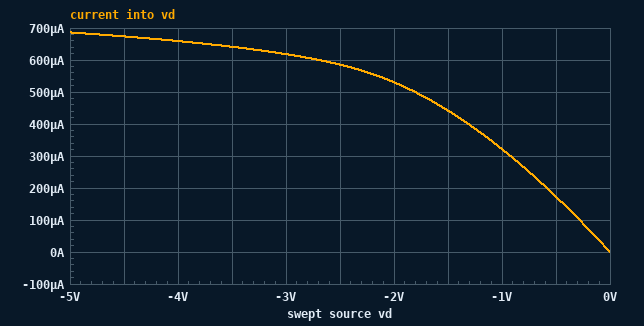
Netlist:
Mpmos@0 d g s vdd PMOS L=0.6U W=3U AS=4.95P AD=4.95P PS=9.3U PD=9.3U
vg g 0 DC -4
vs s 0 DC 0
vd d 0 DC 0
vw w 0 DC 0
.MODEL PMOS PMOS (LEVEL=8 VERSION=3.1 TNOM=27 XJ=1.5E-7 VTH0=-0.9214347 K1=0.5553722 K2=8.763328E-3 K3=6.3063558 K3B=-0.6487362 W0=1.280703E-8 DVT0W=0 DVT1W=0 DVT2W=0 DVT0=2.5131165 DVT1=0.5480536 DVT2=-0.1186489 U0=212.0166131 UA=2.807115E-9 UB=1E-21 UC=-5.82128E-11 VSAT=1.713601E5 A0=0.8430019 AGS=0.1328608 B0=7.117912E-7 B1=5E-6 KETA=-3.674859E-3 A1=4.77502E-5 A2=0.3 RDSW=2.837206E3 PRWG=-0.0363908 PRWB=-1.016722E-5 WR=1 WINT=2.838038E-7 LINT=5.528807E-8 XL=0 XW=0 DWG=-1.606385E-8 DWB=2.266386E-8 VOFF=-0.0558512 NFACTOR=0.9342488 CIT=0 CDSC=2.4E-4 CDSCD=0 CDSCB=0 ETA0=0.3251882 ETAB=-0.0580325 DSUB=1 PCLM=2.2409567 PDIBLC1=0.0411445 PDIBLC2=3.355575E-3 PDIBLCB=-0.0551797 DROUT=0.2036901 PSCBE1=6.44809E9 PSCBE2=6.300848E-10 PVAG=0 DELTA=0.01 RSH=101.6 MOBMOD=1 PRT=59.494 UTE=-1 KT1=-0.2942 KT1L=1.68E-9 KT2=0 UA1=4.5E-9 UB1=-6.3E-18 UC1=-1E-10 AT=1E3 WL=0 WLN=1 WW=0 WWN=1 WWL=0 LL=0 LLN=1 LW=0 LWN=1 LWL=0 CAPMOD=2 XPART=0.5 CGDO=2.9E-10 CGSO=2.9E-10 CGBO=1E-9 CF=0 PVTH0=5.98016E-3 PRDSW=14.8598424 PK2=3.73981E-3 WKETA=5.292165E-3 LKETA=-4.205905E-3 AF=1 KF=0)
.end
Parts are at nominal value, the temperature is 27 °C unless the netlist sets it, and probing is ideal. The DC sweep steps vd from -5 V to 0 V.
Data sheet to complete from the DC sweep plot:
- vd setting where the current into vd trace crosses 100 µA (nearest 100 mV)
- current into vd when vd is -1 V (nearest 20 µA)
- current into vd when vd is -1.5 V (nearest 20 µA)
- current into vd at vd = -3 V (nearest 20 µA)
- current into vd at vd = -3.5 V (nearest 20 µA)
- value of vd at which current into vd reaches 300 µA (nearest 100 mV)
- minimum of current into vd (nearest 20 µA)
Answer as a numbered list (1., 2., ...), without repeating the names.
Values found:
1. -300 mV
2. 320 µA
3. 440 µA
4. 620 µA
5. 640 µA
6. -900 mV
7. 0 A
